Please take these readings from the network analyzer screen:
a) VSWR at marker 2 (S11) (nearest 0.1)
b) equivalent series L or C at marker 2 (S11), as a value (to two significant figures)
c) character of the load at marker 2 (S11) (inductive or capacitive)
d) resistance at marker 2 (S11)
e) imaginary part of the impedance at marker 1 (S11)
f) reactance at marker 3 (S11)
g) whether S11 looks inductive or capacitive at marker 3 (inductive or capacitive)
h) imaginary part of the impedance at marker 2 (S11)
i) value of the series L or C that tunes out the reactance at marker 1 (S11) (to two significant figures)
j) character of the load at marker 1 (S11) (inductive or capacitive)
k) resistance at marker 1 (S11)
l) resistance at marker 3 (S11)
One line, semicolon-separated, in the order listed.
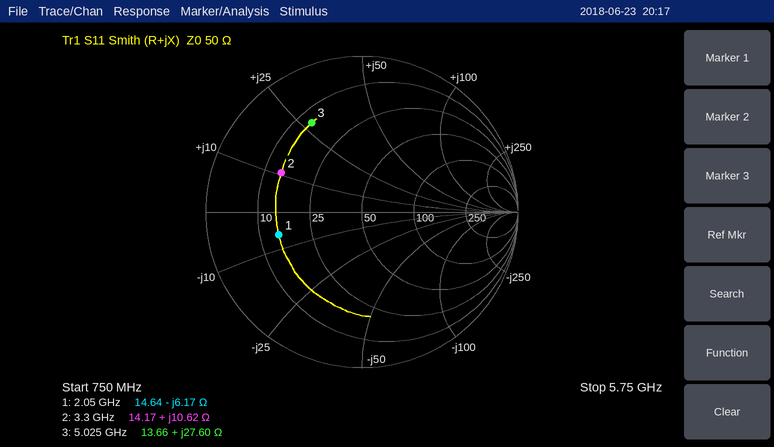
3.7; 510 pH; inductive; 14.17 Ω; -6.17 Ω; +27.60 Ω; inductive; +10.62 Ω; 480 pH; capacitive; 14.64 Ω; 13.66 Ω
